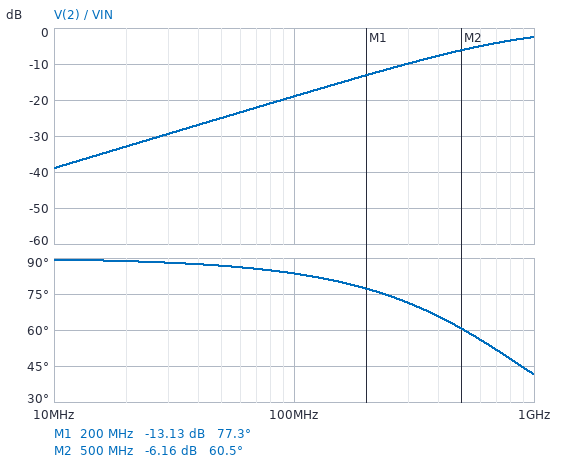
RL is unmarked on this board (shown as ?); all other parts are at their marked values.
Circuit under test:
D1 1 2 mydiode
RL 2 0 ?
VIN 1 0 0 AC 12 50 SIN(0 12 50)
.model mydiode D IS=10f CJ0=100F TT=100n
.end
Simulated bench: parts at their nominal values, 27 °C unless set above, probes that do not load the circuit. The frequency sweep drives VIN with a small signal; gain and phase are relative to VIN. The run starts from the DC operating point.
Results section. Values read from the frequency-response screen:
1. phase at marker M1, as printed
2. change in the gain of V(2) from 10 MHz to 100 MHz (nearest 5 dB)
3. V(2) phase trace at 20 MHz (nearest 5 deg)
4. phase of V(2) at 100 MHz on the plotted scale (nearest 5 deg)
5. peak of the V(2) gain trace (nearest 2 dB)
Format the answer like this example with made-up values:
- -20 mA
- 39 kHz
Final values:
- 77.3 deg
- 20 dB
- 90 deg
- 85 deg
- -2 dB
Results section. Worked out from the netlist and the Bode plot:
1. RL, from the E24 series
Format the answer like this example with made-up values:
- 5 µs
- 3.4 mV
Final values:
- 1.8 kΩ
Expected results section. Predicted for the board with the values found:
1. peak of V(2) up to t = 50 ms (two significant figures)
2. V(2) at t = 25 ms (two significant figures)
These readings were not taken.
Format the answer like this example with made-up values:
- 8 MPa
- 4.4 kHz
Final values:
- 11 V
- 11 V
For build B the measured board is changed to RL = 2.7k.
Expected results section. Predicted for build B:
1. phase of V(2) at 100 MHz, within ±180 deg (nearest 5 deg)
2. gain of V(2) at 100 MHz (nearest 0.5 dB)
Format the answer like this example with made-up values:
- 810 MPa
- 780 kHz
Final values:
- 80 deg
- -15.5 dB
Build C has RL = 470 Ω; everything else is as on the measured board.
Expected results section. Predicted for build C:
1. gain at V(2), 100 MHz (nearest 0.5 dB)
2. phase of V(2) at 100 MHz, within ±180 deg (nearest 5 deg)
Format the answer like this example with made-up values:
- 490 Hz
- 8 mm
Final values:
- -30.5 dB
- 90 deg
